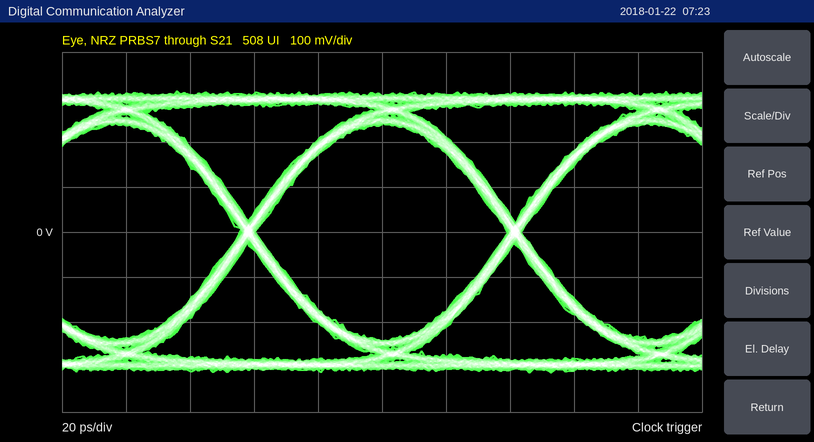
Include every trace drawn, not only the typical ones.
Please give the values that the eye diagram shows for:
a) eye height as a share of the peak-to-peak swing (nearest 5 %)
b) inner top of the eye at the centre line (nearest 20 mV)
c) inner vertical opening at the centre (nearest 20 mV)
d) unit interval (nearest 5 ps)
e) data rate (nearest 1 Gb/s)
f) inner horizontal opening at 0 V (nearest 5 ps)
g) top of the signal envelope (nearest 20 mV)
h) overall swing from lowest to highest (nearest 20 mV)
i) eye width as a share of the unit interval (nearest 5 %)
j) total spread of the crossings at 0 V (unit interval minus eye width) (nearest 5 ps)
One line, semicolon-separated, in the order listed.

75 %; 240 mV; 480 mV; 85 ps; 12 Gb/s; 80 ps; 320 mV; 620 mV; 95 %; 5 ps
